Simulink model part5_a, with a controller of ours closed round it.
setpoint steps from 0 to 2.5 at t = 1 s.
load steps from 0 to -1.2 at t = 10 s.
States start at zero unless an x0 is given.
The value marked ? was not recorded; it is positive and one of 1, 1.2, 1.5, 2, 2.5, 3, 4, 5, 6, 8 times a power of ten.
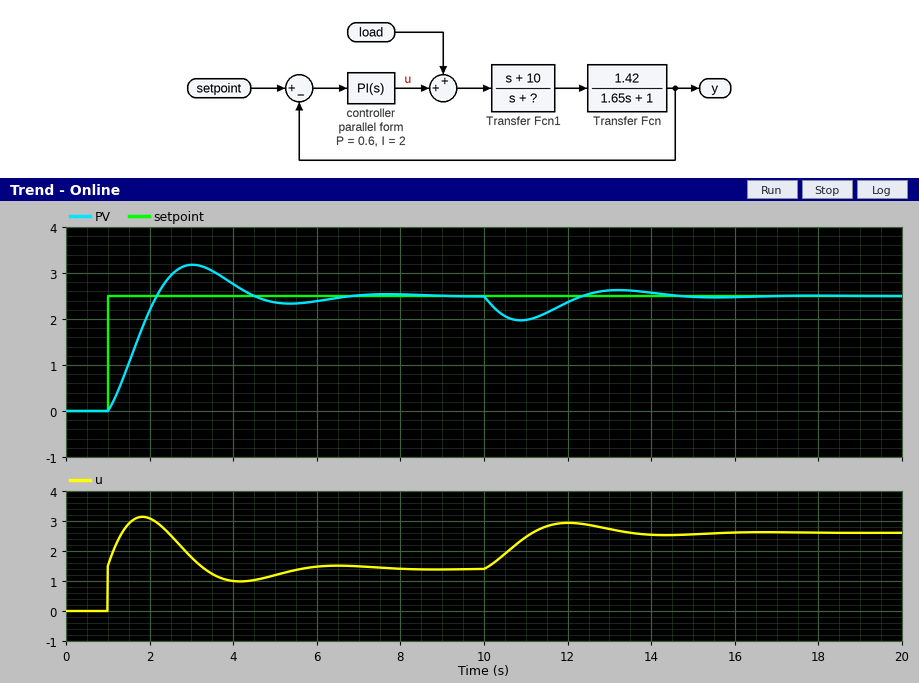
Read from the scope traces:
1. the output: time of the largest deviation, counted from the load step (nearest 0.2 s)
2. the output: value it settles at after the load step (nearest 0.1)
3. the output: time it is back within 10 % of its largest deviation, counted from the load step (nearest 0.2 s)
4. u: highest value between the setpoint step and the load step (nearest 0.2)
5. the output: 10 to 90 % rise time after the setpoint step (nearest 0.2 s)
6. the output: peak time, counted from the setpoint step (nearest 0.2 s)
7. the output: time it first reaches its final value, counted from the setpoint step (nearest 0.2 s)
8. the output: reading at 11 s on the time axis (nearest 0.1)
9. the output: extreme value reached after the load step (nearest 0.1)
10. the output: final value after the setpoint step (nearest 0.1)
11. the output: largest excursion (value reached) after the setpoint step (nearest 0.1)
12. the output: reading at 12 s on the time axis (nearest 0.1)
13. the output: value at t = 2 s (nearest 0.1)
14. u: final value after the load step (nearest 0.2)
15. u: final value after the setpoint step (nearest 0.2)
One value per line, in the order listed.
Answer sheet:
0.8 s
2.5
4.2 s
3.2
0.8 s
2.0 s
1.2 s
2.0
2.0
2.5
3.2
2.4
2.2
2.6
1.4
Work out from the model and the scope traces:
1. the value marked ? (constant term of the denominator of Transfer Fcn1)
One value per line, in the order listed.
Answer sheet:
8
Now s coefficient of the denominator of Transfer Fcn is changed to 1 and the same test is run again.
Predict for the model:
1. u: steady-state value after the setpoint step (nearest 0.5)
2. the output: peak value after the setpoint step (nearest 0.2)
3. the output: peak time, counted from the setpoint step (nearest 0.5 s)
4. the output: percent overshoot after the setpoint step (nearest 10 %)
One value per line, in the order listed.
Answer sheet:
1.5
3.0
1.5 s
20 %
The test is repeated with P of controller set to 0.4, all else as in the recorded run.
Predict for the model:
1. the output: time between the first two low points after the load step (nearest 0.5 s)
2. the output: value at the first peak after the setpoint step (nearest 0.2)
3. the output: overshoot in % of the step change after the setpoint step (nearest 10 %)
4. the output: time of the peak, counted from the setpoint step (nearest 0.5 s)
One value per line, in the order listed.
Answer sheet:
4.5 s
3.4
30 %
2.0 s
